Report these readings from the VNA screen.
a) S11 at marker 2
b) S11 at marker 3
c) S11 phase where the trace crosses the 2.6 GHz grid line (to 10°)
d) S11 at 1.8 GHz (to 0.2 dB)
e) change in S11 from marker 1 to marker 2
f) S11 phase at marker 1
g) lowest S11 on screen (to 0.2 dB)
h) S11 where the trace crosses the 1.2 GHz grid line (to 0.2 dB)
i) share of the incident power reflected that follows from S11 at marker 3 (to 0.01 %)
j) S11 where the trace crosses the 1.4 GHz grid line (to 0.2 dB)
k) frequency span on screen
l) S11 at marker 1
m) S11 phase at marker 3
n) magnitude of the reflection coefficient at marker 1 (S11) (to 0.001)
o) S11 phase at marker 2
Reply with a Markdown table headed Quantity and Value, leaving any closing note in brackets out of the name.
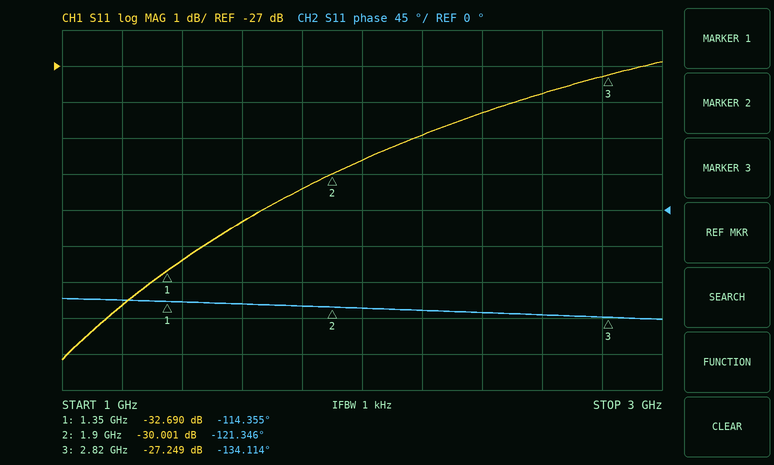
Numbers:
| Quantity | Value |
|---|---|
| S11 at marker 2 | -30.001 dB |
| S11 at marker 3 | -27.249 dB |
| S11 phase where the trace crosses the 2.6 GHz grid line | -130° |
| S11 at 1.8 GHz | -30.4 dB |
| change in S11 from marker 1 to marker 2 | 2.689 dB |
| S11 phase at marker 1 | -114.355° |
| lowest S11 on screen | -35.2 dB |
| S11 where the trace crosses the 1.2 GHz grid line | -33.6 dB |
| share of the incident power reflected that follows from S11 at marker 3 | 0.19 % |
| S11 where the trace crosses the 1.4 GHz grid line | -32.4 dB |
| frequency span on screen | 2 GHz |
| S11 at marker 1 | -32.690 dB |
| S11 phase at marker 3 | -134.114° |
| magnitude of the reflection coefficient at marker 1 (S11) | 0.023 |
| S11 phase at marker 2 | -121.346° |
